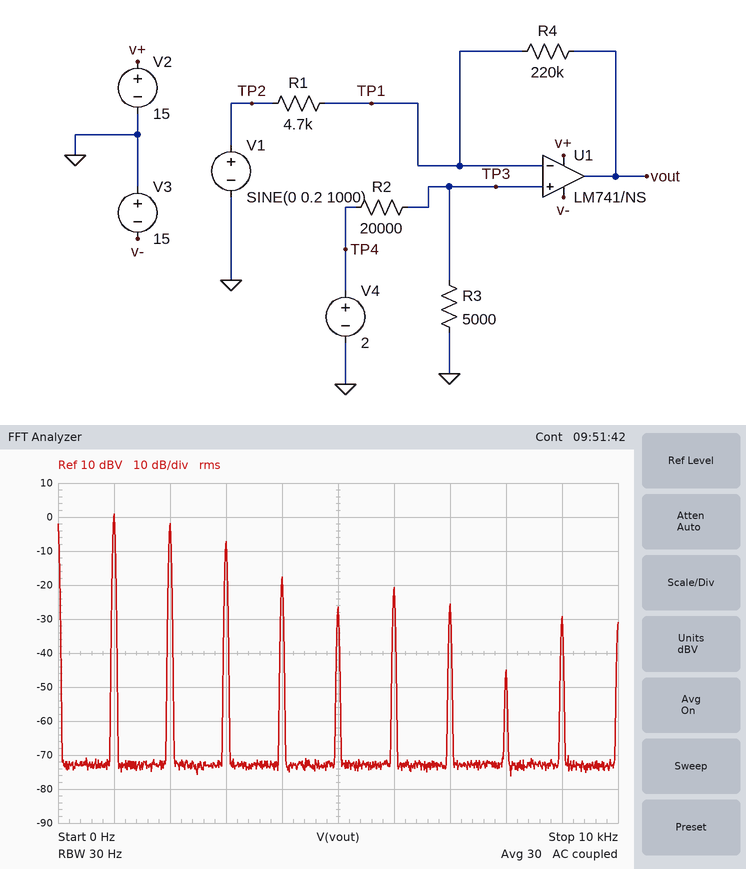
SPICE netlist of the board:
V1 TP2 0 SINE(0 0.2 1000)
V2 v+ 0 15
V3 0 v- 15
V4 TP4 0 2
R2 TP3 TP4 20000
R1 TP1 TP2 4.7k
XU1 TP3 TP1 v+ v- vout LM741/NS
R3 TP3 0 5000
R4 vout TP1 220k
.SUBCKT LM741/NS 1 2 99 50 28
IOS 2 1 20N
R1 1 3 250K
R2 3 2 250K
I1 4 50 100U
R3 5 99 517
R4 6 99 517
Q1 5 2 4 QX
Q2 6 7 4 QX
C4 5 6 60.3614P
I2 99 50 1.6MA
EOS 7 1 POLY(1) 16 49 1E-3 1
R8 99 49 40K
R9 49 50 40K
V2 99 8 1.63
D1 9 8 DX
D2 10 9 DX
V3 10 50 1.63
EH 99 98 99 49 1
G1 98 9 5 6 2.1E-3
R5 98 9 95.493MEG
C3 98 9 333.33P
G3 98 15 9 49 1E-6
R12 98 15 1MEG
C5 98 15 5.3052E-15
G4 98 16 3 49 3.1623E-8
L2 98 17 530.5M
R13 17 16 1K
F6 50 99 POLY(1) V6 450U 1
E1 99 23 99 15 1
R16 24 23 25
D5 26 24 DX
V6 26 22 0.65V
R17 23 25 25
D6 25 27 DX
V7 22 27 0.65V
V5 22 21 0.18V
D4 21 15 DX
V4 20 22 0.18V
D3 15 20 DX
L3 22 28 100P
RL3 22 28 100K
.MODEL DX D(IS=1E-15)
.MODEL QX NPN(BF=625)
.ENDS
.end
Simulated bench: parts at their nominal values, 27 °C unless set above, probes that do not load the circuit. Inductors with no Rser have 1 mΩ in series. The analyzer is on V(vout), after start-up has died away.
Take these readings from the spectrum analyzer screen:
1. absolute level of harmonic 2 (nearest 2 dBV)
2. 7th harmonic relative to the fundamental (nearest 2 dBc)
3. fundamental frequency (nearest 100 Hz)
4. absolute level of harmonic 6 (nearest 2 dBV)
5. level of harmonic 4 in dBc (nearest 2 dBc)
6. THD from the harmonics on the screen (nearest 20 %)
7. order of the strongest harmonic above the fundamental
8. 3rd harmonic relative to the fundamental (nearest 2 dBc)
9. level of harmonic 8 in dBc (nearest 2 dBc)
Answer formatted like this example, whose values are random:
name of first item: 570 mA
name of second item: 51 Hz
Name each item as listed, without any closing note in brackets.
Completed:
absolute level of harmonic 2: -2 dBV
7th harmonic relative to the fundamental: -26 dBc
fundamental frequency: 1.0 kHz
absolute level of harmonic 6: -20 dBV
level of harmonic 4 in dBc: -18 dBc
THD from the harmonics on the screen: 80 %
order of the strongest harmonic above the fundamental: 2
3rd harmonic relative to the fundamental: -8 dBc
level of harmonic 8 in dBc: -46 dBc
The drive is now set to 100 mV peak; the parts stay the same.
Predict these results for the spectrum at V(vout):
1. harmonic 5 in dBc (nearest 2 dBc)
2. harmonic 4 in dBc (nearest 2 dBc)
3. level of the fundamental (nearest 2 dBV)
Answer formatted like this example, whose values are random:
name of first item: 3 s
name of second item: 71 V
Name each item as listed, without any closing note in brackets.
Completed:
harmonic 5 in dBc: -22 dBc
harmonic 4 in dBc: -16 dBc
level of the fundamental: -40 dBV
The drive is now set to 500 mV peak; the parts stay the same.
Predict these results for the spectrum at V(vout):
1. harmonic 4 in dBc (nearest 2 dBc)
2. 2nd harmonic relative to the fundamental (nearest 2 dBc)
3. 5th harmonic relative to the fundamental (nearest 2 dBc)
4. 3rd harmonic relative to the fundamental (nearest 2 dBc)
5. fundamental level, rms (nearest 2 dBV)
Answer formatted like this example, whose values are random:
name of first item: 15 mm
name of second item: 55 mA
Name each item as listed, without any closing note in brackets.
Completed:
harmonic 4 in dBc: -22 dBc
2nd harmonic relative to the fundamental: -6 dBc
5th harmonic relative to the fundamental: -24 dBc
3rd harmonic relative to the fundamental: -18 dBc
fundamental level, rms: 16 dBV
